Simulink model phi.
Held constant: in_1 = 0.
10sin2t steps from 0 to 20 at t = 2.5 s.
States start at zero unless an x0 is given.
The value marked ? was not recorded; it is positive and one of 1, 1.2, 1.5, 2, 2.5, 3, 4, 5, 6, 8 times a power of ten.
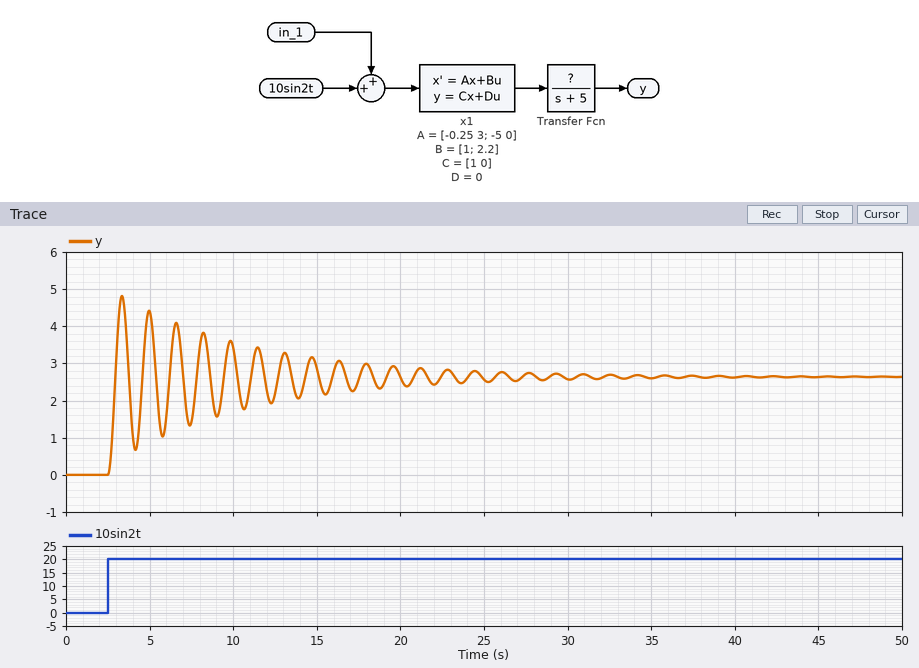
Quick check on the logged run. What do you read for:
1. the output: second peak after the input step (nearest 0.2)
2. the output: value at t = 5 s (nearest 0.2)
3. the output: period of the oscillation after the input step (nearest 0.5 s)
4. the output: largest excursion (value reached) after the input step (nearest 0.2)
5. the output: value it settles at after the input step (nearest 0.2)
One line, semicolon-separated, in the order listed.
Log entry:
4.4; 4.4; 1.5 s; 4.8; 2.6
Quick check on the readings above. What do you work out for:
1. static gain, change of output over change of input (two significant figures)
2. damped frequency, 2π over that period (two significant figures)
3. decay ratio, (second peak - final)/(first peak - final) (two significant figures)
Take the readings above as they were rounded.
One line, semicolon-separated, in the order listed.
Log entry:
0.13; 4.2 rad/s; 0.82
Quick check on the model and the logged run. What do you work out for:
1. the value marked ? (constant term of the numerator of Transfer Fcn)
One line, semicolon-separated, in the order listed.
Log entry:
1.5
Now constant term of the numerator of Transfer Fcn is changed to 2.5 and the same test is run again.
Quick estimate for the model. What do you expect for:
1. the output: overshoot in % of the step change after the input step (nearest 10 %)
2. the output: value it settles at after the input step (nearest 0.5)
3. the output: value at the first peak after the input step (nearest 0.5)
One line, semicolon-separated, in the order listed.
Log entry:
80 %; 4.5; 8.0
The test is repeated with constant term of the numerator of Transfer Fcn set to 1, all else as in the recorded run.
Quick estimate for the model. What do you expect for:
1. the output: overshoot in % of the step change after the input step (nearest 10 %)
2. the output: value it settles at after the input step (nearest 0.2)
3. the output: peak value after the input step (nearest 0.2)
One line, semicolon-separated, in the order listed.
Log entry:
80 %; 1.8; 3.2
